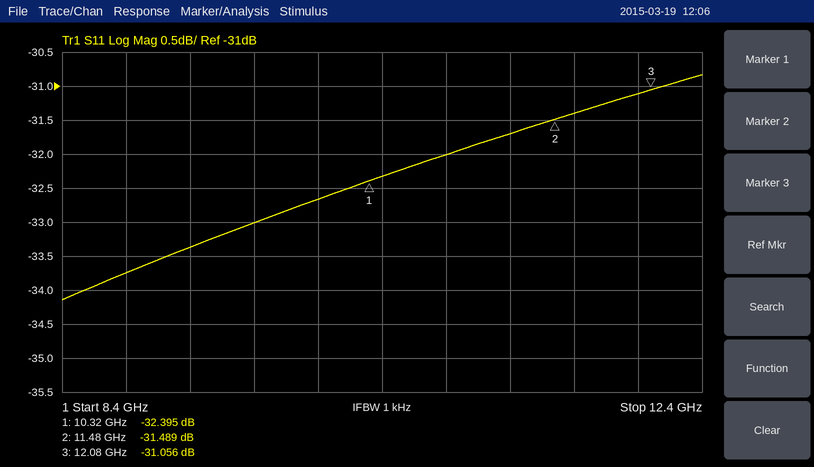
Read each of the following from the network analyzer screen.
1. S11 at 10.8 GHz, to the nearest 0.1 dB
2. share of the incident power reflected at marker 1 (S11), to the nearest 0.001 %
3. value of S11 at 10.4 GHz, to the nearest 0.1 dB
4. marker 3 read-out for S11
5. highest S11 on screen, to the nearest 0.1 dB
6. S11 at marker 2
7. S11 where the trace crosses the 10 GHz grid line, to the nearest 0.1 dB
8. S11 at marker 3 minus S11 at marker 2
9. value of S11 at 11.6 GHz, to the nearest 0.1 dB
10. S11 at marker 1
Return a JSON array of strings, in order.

["-32.0 dB", "0.058 %", "-32.3 dB", "-31.056 dB", "-30.8 dB", "-31.489 dB", "-32.7 dB", "0.433 dB", "-31.4 dB", "-32.395 dB"]
